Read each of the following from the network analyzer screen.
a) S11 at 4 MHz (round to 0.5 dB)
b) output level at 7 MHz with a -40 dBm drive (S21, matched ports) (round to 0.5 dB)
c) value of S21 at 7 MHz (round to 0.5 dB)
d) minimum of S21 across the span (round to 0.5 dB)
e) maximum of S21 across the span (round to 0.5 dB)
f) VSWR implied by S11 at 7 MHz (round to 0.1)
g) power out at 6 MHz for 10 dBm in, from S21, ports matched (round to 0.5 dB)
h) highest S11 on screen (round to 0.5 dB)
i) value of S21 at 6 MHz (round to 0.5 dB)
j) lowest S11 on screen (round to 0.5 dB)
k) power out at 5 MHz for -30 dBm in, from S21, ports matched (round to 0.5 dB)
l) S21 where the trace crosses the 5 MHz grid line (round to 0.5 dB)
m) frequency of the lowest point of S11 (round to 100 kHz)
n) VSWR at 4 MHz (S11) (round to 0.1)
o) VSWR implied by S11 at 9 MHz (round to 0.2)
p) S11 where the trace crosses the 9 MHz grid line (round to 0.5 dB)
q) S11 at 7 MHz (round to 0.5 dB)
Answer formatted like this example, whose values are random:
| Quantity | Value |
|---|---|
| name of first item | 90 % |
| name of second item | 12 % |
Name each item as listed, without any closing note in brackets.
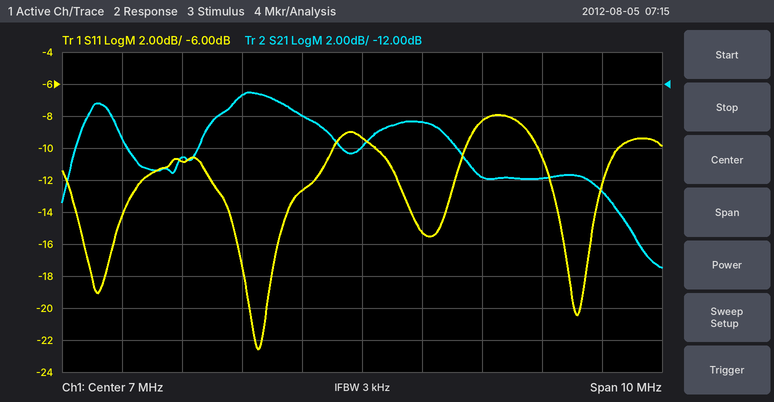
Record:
| Quantity | Value |
|---|---|
| S11 at 4 MHz | -11.0 dB |
| output level at 7 MHz with a -40 dBm drive (S21, matched ports) | -56.0 dBm |
| value of S21 at 7 MHz | -16.0 dB |
| minimum of S21 across the span | -23.5 dB |
| maximum of S21 across the span | -12.5 dB |
| VSWR implied by S11 at 7 MHz | 2.0 |
| power out at 6 MHz for 10 dBm in, from S21, ports matched | -4.0 dBm |
| highest S11 on screen | -8.0 dB |
| value of S21 at 6 MHz | -14.0 dB |
| lowest S11 on screen | -22.5 dB |
| power out at 5 MHz for -30 dBm in, from S21, ports matched | -42.5 dBm |
| S21 where the trace crosses the 5 MHz grid line | -12.5 dB |
| frequency of the lowest point of S11 | 5.3 MHz |
| VSWR at 4 MHz (S11) | 1.8 |
| VSWR implied by S11 at 9 MHz | 2.2 |
| S11 where the trace crosses the 9 MHz grid line | -8.5 dB |
| S11 at 7 MHz | -9.5 dB |
